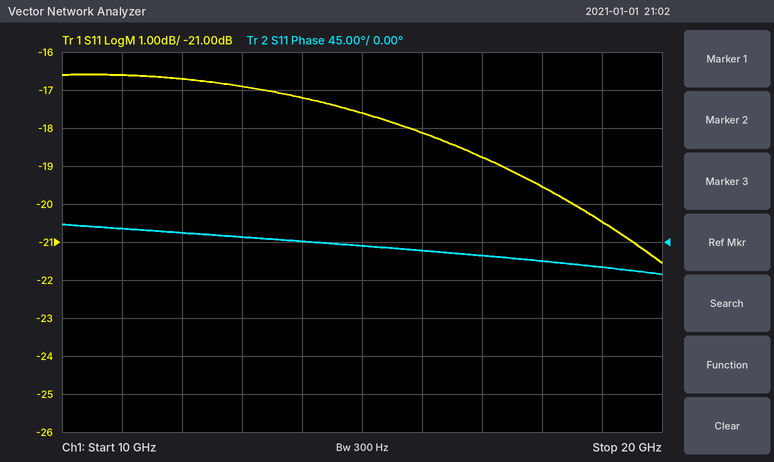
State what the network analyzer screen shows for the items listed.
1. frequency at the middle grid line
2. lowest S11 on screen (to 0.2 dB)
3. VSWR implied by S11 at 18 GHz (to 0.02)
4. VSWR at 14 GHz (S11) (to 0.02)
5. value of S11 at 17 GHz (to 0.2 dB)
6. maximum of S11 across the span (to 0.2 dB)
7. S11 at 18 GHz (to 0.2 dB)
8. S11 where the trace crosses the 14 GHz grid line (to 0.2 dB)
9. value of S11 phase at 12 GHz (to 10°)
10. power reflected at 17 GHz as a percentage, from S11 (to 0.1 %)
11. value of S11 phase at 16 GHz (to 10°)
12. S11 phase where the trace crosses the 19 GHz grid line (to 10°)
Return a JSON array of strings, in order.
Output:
["15 GHz", "-21.6 dB", "1.24", "1.32", "-18.8 dB", "-16.6 dB", "-19.6 dB", "-17.2 dB", "10°", "1.3 %", "-10°", "-30°"]
